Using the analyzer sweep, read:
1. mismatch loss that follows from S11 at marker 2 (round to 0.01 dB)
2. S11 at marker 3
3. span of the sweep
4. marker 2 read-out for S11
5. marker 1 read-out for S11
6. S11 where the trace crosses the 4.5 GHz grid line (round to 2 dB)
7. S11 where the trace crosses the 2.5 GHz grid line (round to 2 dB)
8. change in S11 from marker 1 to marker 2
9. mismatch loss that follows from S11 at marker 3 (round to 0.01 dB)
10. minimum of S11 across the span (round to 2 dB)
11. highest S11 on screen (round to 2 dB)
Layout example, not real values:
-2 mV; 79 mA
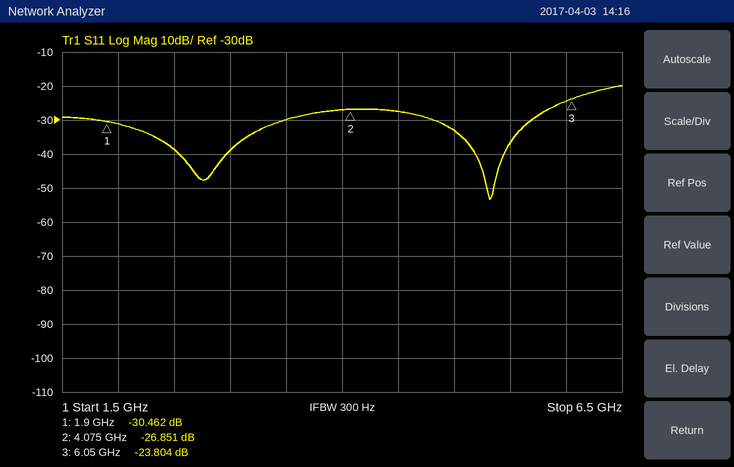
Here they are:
0.01 dB; -23.804 dB; 5 GHz; -26.851 dB; -30.462 dB; -28 dB; -38 dB; 3.611 dB; 0.02 dB; -54 dB; -20 dB
